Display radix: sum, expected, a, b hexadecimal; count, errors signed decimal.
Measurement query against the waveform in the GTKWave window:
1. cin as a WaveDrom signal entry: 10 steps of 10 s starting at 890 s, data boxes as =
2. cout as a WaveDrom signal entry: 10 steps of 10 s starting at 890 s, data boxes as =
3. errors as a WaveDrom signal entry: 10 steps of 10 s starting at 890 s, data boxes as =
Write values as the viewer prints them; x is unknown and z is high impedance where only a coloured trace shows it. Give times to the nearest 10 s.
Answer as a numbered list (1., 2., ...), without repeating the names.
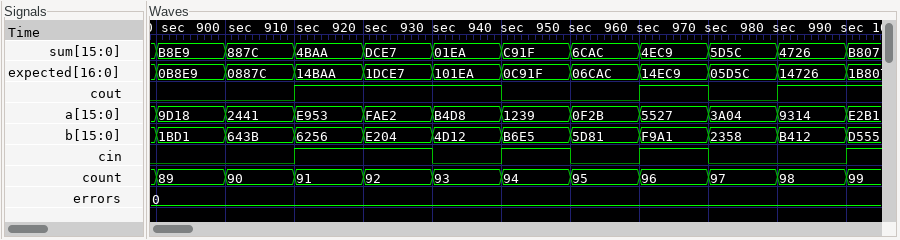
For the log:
1. {name: 'cin', wave: '0.1.01010.'}
2. {name: 'cout', wave: '0.1..0.101'}
3. {name: 'errors', wave: '=.........', data: '0'}
